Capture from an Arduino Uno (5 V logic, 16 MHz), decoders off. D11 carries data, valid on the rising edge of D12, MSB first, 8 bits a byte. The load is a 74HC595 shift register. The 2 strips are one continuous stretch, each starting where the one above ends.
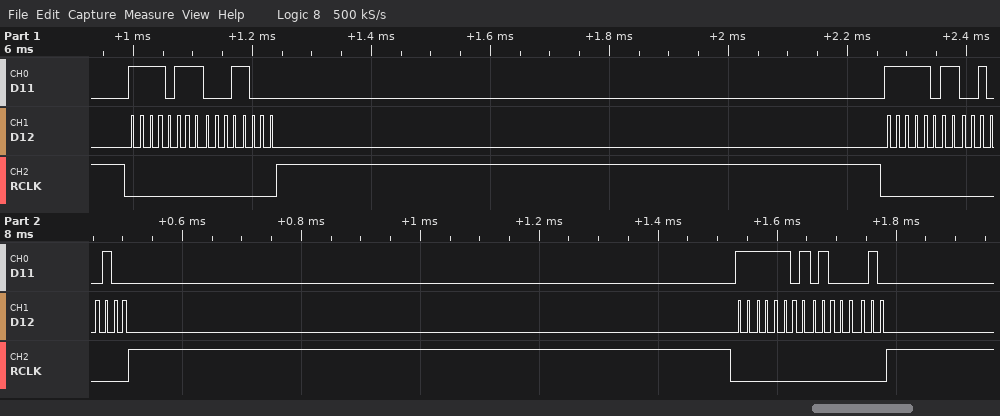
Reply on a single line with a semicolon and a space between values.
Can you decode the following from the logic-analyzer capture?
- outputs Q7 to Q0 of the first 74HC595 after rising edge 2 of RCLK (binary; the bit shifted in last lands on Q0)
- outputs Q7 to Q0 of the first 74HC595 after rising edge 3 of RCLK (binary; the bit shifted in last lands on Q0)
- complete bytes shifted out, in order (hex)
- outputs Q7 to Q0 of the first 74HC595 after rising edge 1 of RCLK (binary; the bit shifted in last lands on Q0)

00100100; 01000010; F7 18 FB 24 FD 42; 00011000
